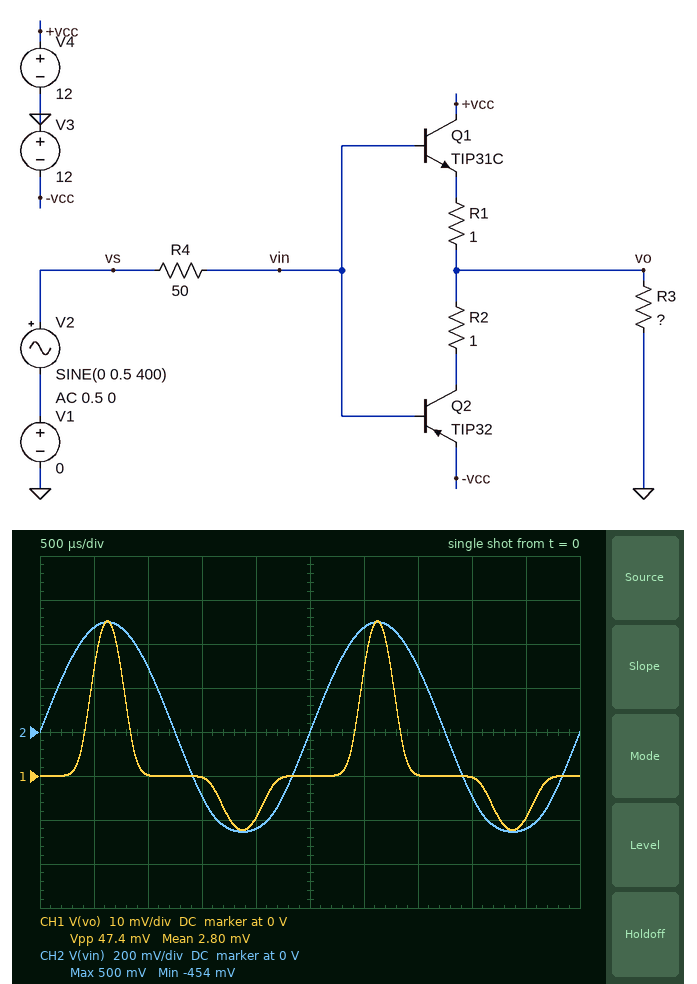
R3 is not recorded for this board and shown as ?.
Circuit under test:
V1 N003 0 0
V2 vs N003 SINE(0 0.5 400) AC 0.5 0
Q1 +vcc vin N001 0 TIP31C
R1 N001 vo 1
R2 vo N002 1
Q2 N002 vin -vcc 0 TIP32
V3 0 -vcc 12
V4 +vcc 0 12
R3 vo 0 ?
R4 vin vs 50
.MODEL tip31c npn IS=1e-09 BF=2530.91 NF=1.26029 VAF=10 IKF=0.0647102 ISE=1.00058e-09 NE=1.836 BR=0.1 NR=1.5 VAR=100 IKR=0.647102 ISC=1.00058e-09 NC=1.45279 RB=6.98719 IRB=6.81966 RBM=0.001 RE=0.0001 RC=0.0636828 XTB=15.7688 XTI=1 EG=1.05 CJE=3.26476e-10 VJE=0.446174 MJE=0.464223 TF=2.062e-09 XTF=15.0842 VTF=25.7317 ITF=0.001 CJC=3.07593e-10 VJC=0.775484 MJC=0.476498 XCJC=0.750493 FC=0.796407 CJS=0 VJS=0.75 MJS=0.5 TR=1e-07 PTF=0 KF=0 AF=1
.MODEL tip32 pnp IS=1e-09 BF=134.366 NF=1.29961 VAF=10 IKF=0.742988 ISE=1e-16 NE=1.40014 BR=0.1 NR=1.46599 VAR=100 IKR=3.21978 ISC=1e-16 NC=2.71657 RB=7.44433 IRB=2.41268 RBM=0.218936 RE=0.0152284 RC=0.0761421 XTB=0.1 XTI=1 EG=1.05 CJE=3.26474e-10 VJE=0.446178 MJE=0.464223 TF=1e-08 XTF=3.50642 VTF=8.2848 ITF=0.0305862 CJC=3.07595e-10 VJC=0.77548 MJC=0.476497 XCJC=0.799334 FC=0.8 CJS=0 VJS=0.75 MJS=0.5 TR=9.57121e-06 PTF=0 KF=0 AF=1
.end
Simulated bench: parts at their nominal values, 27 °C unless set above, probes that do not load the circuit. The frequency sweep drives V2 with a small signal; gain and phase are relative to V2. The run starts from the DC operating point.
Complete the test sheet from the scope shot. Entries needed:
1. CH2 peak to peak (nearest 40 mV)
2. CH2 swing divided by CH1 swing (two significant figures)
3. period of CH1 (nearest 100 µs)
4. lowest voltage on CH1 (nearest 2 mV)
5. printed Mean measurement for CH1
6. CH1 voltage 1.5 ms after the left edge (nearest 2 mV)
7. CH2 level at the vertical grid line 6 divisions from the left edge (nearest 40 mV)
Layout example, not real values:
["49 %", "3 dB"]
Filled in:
["960 mV", "20", "2.5 ms", "-12 mV", "2.80 mV", "0 V", "480 mV"]
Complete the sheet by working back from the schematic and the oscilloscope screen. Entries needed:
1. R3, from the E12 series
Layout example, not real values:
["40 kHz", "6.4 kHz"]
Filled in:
["12 Ω"]
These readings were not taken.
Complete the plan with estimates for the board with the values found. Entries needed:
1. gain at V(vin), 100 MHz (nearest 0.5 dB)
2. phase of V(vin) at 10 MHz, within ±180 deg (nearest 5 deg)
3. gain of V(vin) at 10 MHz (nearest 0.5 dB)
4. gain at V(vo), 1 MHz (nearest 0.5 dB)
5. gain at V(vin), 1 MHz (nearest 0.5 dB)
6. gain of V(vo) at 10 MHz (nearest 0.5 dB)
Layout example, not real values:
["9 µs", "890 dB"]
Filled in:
["-15.5 dB", "-45 deg", "-8.5 dB", "-27.0 dB", "-0.5 dB", "-16.5 dB"]
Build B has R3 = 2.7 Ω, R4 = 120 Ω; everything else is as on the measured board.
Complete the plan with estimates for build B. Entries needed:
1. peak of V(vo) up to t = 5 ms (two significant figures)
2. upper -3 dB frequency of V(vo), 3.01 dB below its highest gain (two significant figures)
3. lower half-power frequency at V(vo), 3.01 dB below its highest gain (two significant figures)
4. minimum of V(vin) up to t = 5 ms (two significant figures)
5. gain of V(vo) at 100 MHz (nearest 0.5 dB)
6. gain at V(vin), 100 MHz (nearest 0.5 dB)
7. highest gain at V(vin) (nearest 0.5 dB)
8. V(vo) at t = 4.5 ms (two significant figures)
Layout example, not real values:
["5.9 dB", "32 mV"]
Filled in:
["13 mV", "410 MHz", "1.6 MHz", "-430 mV", "-35.5 dB", "-27.0 dB", "0 dB", "-1.5 mV"]
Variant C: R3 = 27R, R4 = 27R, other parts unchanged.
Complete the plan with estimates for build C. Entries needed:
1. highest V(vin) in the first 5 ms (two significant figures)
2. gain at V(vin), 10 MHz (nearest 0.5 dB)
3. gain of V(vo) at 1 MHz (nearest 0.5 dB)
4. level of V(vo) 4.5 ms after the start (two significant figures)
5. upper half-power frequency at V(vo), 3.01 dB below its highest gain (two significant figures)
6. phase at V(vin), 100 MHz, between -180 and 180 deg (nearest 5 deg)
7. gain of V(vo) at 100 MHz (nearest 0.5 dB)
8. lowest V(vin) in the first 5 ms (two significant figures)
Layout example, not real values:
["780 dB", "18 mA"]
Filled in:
["500 mV", "-4.5 dB", "-19.5 dB", "-23 mV", "87 MHz", "-40 deg", "-11.5 dB", "-470 mV"]
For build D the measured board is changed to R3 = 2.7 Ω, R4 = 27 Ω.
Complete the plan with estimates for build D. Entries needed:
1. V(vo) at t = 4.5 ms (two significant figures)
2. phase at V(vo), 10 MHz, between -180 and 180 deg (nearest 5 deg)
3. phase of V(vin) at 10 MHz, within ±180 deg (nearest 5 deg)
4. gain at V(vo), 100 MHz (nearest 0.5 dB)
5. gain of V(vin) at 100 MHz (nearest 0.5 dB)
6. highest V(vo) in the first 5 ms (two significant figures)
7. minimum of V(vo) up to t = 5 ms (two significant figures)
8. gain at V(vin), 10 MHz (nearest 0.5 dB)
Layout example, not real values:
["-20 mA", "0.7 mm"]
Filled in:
["-3.0 mV", "30 deg", "-45 deg", "-23.5 dB", "-15.0 dB", "14 mV", "-4.0 mV", "-5.0 dB"]
